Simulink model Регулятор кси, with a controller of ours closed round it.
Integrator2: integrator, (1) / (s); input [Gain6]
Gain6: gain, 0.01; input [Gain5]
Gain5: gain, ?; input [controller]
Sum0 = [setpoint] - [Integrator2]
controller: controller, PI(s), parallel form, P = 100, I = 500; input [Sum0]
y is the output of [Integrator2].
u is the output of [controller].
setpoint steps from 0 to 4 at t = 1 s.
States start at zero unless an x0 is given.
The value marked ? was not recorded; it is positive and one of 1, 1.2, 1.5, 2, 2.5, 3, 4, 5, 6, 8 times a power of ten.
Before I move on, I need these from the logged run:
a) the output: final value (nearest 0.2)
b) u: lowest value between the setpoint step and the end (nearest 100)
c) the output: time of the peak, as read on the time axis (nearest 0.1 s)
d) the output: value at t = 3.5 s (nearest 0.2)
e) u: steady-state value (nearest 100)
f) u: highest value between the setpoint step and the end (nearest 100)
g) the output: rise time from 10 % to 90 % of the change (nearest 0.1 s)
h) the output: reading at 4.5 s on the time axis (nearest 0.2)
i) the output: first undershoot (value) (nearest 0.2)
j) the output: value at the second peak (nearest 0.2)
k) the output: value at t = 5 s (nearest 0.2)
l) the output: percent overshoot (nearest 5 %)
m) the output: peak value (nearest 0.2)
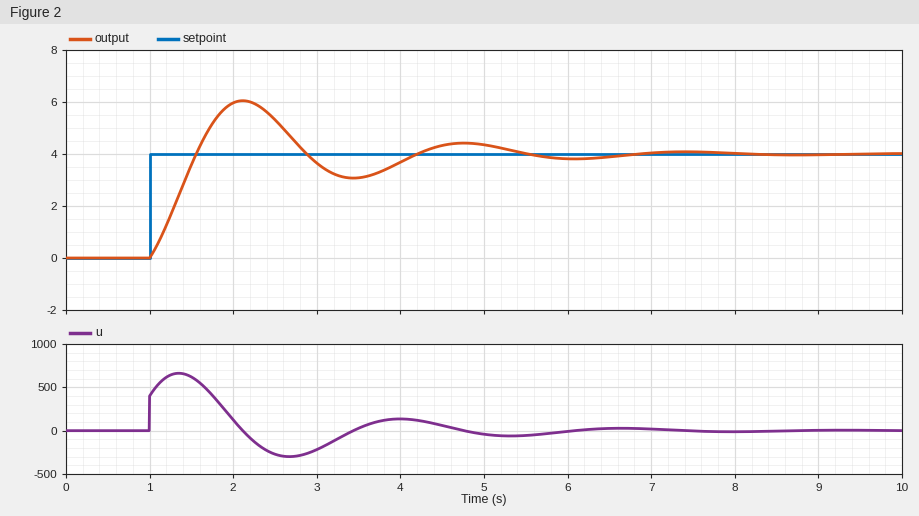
4.0
-300
2.1 s
3.0
0
700
0.4 s
4.4
3.0
4.4
4.4
50 %
6.0
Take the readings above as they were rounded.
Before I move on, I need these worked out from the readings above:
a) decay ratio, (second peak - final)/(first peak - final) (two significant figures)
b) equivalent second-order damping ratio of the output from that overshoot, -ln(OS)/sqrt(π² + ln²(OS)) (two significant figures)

0.20
0.22
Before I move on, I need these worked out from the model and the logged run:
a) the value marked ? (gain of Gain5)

1.2
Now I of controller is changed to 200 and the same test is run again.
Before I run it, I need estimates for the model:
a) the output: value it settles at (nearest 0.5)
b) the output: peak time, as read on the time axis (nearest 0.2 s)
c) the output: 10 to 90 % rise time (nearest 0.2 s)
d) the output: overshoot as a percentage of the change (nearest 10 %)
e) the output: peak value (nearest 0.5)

4.0
2.6 s
0.6 s
40 %
5.5
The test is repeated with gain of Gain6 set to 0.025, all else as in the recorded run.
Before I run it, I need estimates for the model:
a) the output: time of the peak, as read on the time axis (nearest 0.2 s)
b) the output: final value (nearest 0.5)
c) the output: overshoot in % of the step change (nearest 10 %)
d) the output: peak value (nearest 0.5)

1.6 s
4.0
40 %
5.5
